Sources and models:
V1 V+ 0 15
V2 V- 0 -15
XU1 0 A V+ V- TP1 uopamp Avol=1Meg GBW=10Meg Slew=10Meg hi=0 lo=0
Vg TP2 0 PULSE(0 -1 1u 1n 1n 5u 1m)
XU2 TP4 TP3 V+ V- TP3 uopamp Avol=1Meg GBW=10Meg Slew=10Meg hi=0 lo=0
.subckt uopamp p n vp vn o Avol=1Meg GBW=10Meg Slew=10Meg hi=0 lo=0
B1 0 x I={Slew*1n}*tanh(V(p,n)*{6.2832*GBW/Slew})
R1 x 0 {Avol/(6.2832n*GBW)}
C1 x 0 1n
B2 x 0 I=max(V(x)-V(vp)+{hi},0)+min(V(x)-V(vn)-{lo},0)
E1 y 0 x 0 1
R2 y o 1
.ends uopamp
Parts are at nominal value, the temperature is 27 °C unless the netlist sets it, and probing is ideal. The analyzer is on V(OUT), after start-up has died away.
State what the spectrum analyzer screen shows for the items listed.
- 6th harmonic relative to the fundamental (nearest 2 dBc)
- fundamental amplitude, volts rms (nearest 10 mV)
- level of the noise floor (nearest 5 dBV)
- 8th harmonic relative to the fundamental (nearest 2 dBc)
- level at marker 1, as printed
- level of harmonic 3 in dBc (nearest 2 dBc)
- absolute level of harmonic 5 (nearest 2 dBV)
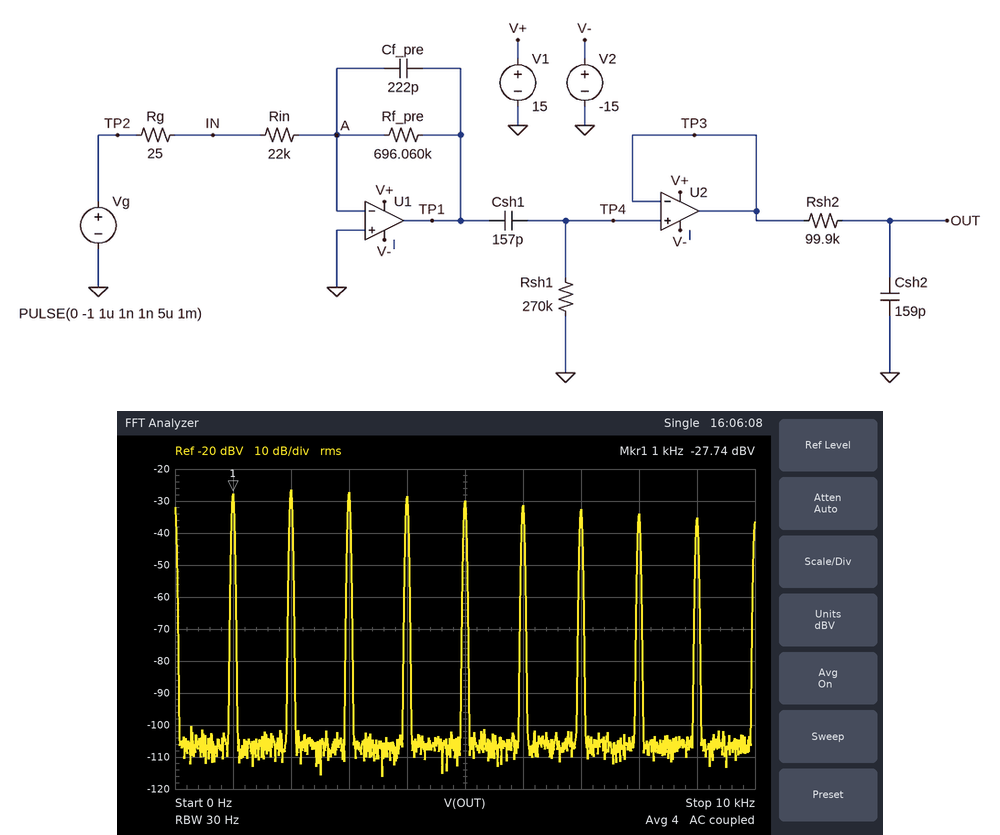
-4 dBc
40 mV
-105 dBV
-6 dBc
-27.74 dBV
0 dBc
-30 dBV
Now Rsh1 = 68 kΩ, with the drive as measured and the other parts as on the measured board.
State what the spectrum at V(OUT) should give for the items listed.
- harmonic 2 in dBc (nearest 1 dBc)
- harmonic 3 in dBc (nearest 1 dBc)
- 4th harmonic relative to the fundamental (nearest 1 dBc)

2 dBc
2 dBc
2 dBc
